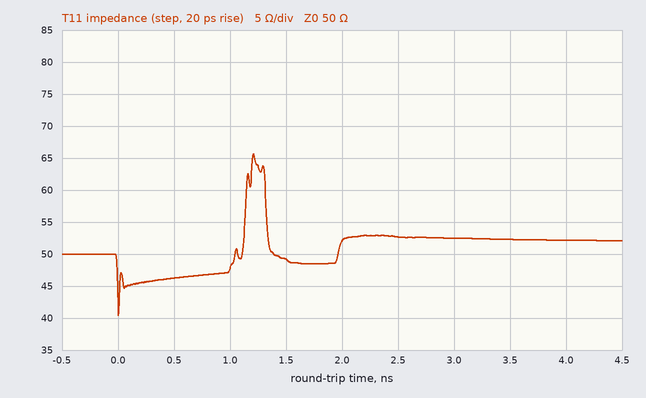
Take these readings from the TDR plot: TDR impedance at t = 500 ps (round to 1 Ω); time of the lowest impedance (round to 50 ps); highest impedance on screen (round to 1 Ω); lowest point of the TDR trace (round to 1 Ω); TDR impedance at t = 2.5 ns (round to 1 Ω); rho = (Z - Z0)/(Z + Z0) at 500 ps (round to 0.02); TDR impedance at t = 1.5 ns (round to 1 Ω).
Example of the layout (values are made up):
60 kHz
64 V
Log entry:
46 Ω
0 ps
66 Ω
40 Ω
53 Ω
-0.04
49 Ω
